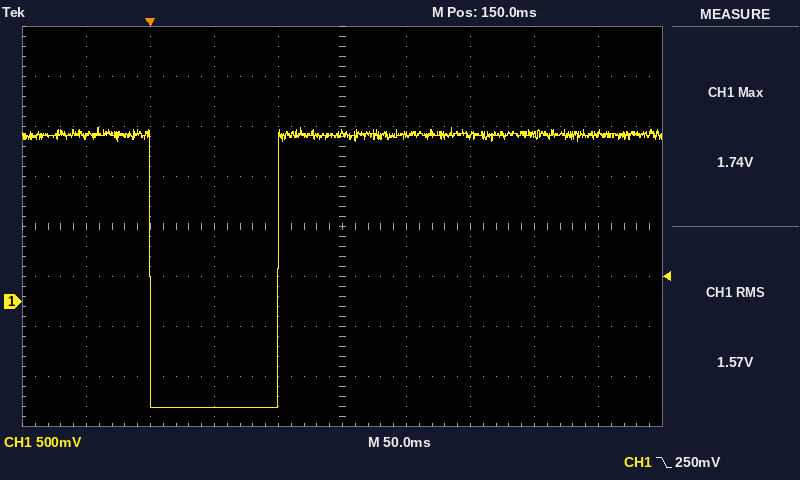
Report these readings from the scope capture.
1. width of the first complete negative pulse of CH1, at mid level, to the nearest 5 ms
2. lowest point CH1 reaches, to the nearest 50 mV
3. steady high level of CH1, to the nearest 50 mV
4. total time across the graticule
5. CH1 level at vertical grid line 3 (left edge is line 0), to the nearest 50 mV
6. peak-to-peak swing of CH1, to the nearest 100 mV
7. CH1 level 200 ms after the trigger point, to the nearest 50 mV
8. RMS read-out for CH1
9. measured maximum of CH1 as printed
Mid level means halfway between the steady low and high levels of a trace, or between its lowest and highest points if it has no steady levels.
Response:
100 ms
-1.05 V
1.65 V
500 ms
-1.05 V
2.80 V
1.65 V
1.57 V
1.74 V
